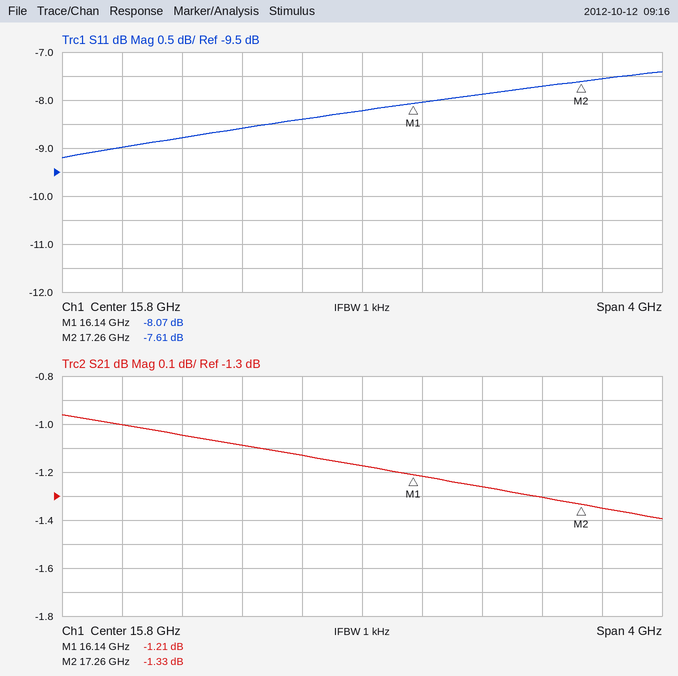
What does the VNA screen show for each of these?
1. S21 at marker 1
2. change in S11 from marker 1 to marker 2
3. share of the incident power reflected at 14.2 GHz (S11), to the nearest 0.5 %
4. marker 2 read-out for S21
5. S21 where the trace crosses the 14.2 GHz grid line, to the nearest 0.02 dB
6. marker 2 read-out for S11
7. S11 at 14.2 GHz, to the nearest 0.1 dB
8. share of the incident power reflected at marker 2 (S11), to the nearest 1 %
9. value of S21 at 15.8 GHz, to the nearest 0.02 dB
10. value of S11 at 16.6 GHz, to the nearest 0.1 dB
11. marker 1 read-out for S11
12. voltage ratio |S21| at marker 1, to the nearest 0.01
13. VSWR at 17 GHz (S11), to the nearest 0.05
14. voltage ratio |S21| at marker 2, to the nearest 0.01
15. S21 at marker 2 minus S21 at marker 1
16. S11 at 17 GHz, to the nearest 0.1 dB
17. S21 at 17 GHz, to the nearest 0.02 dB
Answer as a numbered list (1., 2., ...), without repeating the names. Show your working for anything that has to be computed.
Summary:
1. -1.21 dB
2. -7.61 − (-8.07) = 0.46 dB
3. 10^(-9/10) ≈ 12.6 %, so 12.5 % to the nearest 0.5 %
4. -1.33 dB
5. -1.00 dB
6. -7.61 dB
7. -9.0 dB
8. 10^(-7.61/10) ≈ 17 %
9. -1.18 dB
10. -7.9 dB
11. -8.07 dB
12. 10^(-1.21/20) ≈ 0.87
13. |Γ| = 10^(-7.7/20) = 0.4121; VSWR = (1 + 0.4121)/(1 − 0.4121) ≈ 2.40
14. 10^(-1.33/20) ≈ 0.86
15. -1.33 − (-1.21) = -0.12 dB
16. -7.7 dB
17. -1.30 dB
